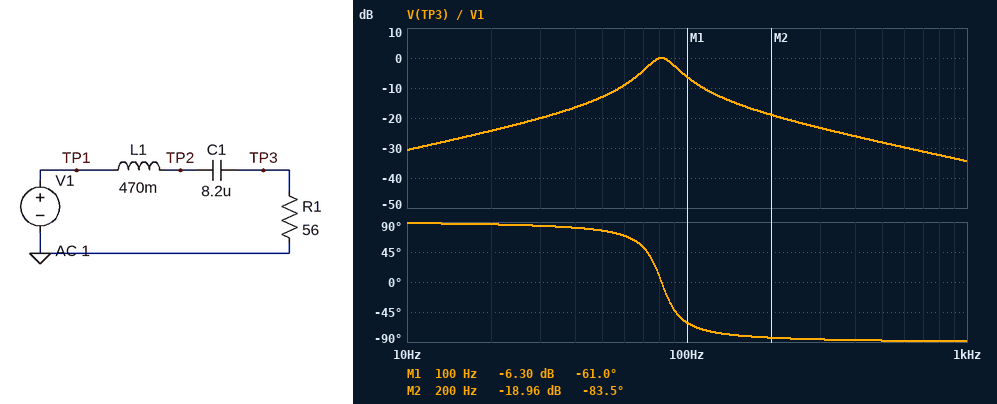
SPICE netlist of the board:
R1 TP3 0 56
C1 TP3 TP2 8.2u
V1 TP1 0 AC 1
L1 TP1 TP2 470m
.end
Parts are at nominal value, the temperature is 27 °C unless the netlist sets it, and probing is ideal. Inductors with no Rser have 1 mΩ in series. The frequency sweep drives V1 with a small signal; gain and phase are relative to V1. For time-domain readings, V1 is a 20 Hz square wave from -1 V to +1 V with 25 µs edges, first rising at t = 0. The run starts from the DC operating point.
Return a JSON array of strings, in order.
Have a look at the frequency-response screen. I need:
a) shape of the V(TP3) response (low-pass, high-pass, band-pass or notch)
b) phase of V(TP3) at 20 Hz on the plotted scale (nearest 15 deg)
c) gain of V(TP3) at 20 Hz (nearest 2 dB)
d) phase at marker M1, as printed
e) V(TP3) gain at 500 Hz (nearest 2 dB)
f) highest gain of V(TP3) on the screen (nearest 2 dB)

["band-pass", "90 deg", "-24 dB", "-61.0 deg", "-28 dB", "0 dB"]
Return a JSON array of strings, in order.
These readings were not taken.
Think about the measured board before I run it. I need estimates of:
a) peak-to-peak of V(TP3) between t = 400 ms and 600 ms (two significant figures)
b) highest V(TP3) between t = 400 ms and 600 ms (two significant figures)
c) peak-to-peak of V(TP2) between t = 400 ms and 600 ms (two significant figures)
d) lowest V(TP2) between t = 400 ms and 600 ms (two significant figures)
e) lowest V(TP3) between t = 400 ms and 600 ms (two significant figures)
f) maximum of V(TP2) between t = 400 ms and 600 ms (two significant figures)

["640 mV", "320 mV", "4.3 V", "-2.2 V", "-320 mV", "2.2 V"]
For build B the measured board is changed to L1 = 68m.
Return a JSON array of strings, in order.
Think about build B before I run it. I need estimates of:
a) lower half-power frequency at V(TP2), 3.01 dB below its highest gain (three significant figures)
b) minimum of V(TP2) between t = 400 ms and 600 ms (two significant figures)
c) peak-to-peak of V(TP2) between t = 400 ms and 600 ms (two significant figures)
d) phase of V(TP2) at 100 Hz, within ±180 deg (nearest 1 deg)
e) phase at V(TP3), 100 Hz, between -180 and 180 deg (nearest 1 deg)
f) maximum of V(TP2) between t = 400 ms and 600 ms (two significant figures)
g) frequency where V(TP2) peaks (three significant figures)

["121 Hz", "-1.9 V", "3.8 V", "-4 deg", "70 deg", "1.9 V", "198 Hz"]
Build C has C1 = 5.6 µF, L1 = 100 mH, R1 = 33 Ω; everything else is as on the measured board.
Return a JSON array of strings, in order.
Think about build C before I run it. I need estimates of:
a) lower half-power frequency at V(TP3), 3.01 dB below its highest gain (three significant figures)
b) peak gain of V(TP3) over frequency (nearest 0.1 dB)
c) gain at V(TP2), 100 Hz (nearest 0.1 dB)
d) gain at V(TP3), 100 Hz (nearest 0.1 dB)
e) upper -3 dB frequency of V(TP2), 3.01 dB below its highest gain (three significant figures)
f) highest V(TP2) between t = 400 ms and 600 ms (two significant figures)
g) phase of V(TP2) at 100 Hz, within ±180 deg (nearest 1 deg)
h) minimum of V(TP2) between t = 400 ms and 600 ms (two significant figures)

["188 Hz", "0 dB", "2.1 dB", "-16.6 dB", "235 Hz", "2.4 V", "-2 deg", "-2.4 V"]
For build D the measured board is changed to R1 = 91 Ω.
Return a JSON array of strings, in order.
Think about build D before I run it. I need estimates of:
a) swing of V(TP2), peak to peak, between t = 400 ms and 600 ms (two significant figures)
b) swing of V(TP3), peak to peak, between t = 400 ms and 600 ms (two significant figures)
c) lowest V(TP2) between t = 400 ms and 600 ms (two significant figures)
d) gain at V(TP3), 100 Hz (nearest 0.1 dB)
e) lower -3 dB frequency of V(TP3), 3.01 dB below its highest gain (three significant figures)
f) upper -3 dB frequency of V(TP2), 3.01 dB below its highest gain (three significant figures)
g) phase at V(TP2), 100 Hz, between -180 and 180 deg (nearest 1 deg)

["4.2 V", "1.1 V", "-2.1 V", "-3.5 dB", "67.1 Hz", "93.1 Hz", "-113 deg"]
